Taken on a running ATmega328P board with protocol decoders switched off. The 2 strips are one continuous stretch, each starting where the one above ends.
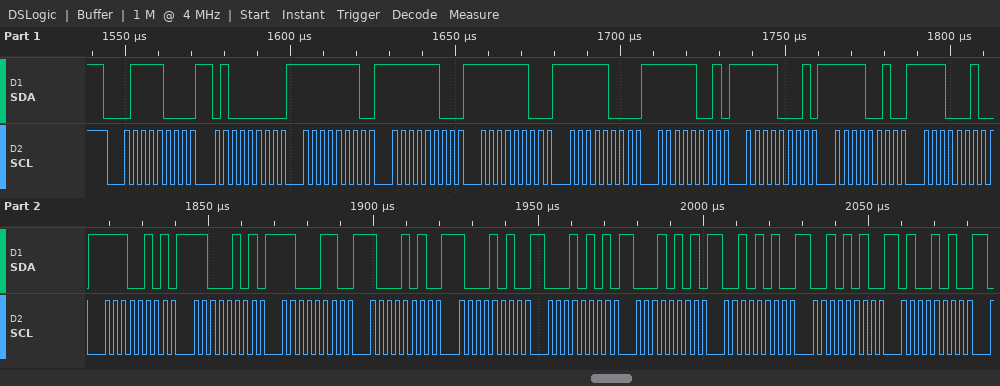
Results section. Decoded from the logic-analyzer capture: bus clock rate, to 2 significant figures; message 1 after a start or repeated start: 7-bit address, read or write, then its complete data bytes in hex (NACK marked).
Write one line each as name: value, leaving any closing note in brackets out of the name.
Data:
bus clock rate, to 2 significant figures: 400 kHz
message 1 after a start or repeated start: 7-bit address, read or write, then its complete data bytes in hex: 0x3C write: 40 FE FC FC F8 F9 F1 F2 E2 E5 C5 C6 8A 8A 15 15 2A 2A 4A
